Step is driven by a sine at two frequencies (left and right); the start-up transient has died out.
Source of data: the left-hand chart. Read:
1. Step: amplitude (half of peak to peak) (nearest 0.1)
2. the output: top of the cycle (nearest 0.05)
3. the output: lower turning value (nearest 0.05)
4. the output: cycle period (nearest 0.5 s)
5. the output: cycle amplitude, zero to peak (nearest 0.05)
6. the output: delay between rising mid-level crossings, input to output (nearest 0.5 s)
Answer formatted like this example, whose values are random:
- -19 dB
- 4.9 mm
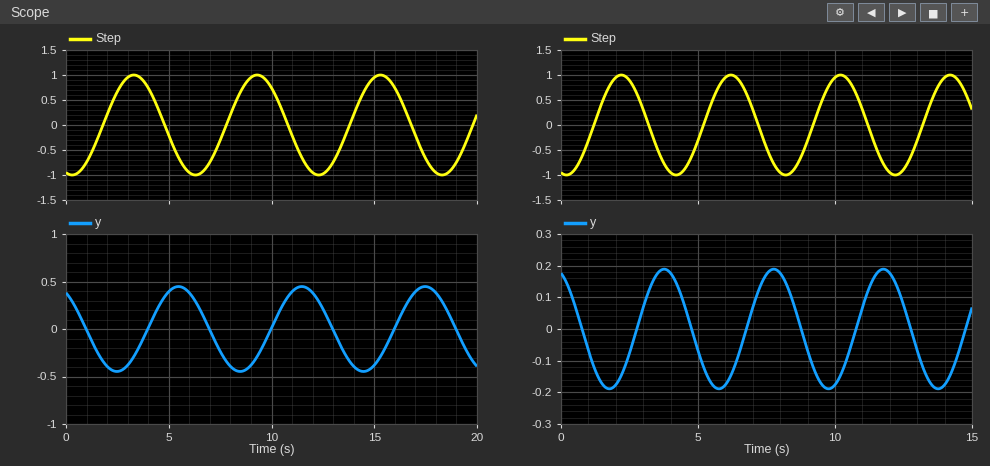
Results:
- 1.0
- 0.45
- -0.45
- 6.0 s
- 0.45
- 2.0 s
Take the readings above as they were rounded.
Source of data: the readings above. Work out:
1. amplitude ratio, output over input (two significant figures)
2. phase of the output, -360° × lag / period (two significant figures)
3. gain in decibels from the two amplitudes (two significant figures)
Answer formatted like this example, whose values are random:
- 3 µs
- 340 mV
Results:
- 0.45
- -120°
- -6.9 dB
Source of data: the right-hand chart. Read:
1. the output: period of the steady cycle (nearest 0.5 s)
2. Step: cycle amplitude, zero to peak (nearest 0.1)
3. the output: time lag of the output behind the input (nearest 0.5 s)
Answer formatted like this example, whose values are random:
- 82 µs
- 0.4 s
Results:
- 4.0 s
- 1.0
- 1.5 s
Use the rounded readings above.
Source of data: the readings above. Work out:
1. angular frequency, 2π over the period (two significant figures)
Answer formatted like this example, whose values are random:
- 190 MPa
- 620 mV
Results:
- 1.6 rad/s
